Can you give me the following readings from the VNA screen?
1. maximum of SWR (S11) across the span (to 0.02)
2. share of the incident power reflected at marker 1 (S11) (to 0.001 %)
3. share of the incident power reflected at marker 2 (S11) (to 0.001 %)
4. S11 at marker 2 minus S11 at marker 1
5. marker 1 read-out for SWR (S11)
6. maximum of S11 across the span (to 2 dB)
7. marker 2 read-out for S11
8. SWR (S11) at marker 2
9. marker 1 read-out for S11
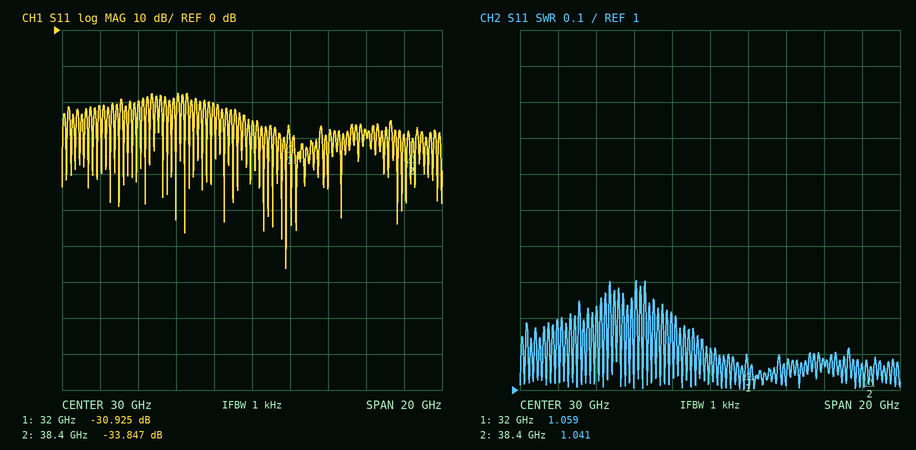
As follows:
1.30
0.081 %
0.041 %
-2.922 dB
1.059
-18 dB
-33.847 dB
1.041
-30.925 dB
